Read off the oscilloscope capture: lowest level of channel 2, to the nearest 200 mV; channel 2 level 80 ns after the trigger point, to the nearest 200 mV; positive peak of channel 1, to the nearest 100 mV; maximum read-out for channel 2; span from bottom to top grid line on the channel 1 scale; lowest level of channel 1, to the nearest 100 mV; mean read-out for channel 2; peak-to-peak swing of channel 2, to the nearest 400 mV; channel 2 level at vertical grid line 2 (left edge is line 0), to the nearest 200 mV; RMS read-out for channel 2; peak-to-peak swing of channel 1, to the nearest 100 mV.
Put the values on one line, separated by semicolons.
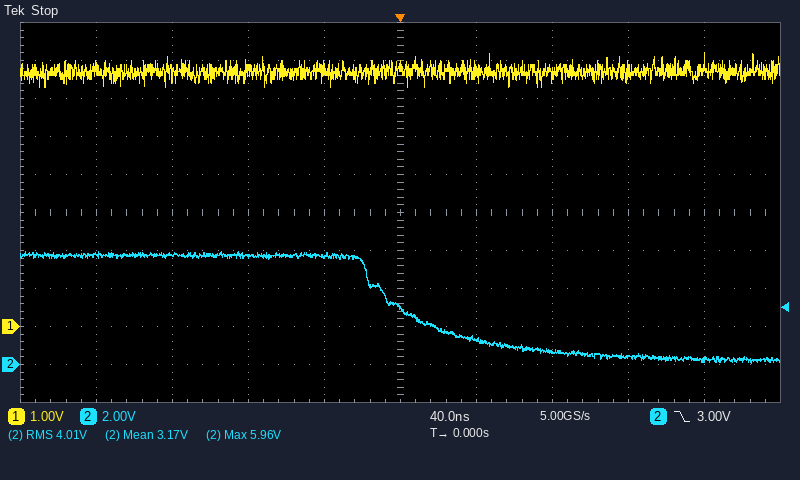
0.0 V; 600 mV; 7.2 V; 5.96 V; 10 V; 6.3 V; 3.17 V; 6.0 V; 5.8 V; 4.01 V; 900 mV
